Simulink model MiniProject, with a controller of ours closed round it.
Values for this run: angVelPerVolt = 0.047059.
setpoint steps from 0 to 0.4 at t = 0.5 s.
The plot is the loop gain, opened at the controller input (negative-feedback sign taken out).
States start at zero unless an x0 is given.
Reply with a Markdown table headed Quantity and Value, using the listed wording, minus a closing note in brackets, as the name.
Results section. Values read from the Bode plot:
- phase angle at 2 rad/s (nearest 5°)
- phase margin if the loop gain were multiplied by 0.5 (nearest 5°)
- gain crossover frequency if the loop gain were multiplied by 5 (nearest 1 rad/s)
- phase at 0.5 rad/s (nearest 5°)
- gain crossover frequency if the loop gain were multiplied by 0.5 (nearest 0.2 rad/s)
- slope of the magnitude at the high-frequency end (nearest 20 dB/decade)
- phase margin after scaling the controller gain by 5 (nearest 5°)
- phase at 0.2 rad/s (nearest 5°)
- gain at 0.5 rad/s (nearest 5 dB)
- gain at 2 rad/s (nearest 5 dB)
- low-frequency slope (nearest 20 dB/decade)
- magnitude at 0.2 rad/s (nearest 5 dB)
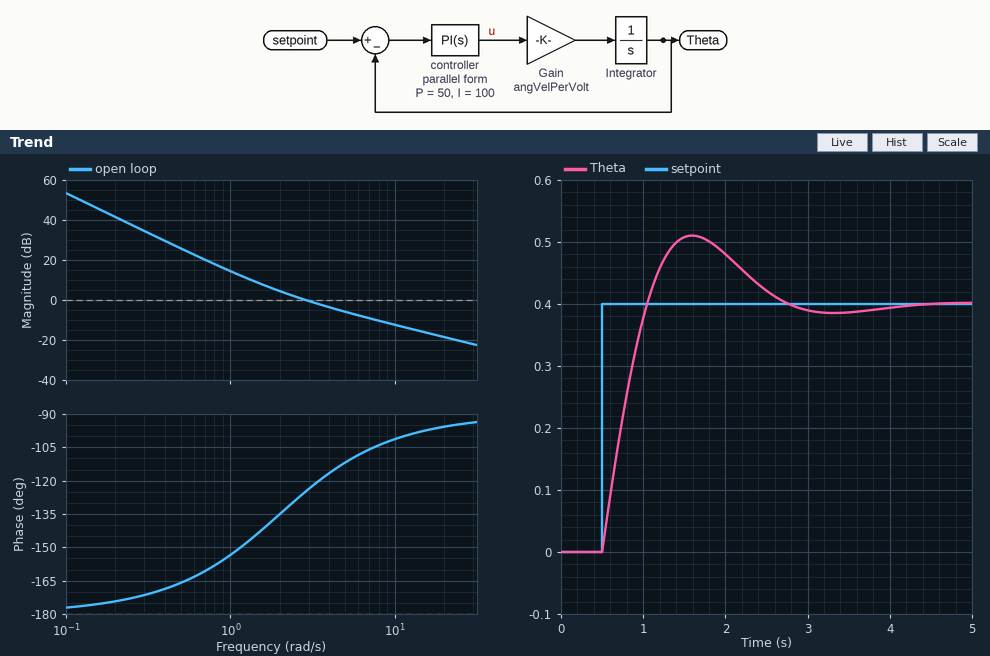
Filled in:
| Quantity | Value |
|---|---|
| phase angle at 2 rad/s | -135° |
| phase margin if the loop gain were multiplied by 0.5 | 40° |
| gain crossover frequency if the loop gain were multiplied by 5 | 12 rad/s |
| phase at 0.5 rad/s | -165° |
| gain crossover frequency if the loop gain were multiplied by 0.5 | 1.8 rad/s |
| slope of the magnitude at the high-frequency end | -20 dB/decade |
| phase margin after scaling the controller gain by 5 | 80° |
| phase at 0.2 rad/s | -175° |
| gain at 0.5 rad/s | 25 dB |
| gain at 2 rad/s | 5 dB |
| low-frequency slope | -40 dB/decade |
| magnitude at 0.2 rad/s | 40 dB |
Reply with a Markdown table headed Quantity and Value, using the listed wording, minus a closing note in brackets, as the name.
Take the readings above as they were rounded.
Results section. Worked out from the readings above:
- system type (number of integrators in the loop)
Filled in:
| Quantity | Value |
|---|---|
| system type | 2 |
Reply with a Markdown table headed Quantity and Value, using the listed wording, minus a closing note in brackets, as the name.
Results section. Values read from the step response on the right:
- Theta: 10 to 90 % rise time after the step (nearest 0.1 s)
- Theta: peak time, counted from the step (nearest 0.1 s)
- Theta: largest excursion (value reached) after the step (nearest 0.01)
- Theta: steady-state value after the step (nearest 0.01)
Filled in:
| Quantity | Value |
|---|---|
| Theta: 10 to 90 % rise time after the step | 0.4 s |
| Theta: peak time, counted from the step | 1.1 s |
| Theta: largest excursion (value reached) after the step | 0.51 |
| Theta: steady-state value after the step | 0.40 |
